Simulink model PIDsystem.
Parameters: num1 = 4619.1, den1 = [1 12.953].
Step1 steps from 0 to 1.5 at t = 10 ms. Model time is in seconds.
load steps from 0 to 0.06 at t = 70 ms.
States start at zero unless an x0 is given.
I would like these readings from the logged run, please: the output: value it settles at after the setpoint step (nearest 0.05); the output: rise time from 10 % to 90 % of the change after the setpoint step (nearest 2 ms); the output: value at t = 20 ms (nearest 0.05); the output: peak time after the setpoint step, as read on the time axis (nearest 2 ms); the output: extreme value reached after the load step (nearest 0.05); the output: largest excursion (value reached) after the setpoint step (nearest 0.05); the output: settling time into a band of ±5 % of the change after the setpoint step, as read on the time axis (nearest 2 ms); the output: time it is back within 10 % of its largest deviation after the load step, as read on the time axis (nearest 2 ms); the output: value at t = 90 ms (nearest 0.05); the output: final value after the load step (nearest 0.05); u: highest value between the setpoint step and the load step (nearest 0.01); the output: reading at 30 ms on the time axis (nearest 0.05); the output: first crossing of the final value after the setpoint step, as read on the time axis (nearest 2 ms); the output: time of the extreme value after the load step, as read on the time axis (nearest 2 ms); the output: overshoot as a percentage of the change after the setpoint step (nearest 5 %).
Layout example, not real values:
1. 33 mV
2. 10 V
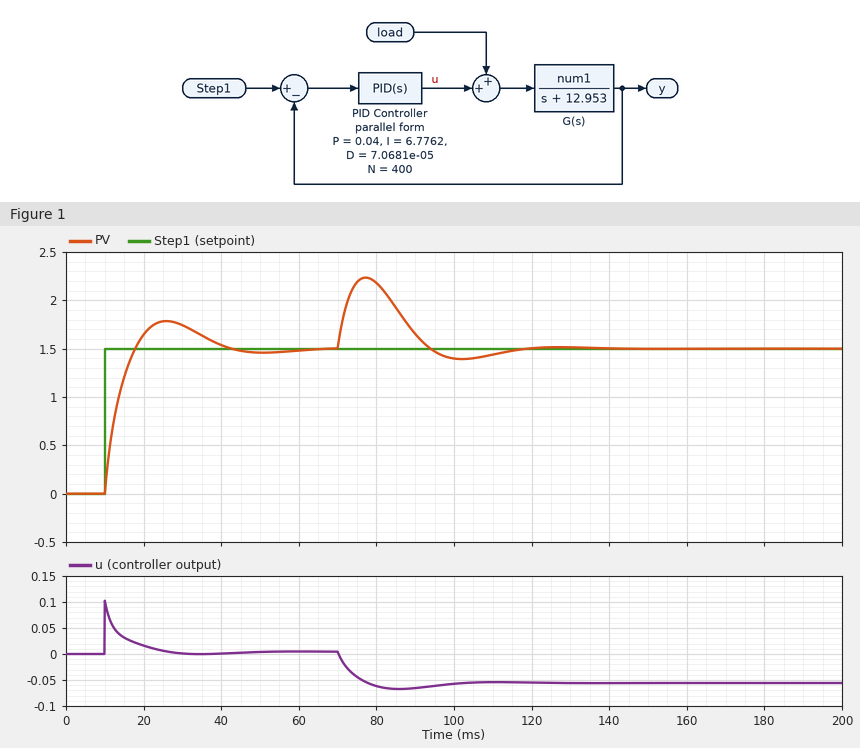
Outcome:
1. 1.50
2. 6 ms
3. 1.65
4. 26 ms
5. 2.25
6. 1.80
7. 38 ms
8. 108 ms
9. 1.65
10. 1.50
11. 0.10
12. 1.75
13. 18 ms
14. 78 ms
15. 20 %
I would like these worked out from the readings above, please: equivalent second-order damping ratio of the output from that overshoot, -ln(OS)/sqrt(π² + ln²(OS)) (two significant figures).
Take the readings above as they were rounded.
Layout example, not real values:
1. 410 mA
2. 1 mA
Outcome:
1. 0.46
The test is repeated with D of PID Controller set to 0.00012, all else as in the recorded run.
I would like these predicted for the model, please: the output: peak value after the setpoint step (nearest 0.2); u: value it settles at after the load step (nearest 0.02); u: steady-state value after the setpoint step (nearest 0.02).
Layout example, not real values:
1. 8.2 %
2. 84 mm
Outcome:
1. 1.8
2. -0.06
3. 0.00
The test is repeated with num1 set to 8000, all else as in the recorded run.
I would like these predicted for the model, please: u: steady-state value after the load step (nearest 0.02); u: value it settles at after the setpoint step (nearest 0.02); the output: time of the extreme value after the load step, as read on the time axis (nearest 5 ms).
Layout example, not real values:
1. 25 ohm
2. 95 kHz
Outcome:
1. -0.06
2. 0.00
3. 75 ms
